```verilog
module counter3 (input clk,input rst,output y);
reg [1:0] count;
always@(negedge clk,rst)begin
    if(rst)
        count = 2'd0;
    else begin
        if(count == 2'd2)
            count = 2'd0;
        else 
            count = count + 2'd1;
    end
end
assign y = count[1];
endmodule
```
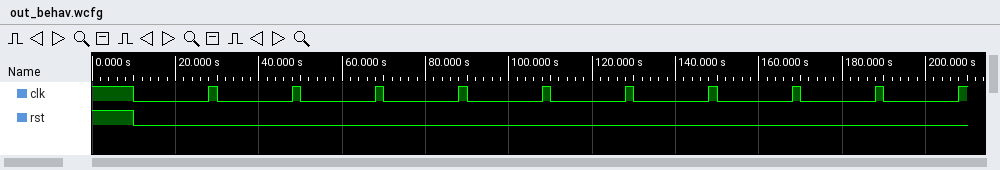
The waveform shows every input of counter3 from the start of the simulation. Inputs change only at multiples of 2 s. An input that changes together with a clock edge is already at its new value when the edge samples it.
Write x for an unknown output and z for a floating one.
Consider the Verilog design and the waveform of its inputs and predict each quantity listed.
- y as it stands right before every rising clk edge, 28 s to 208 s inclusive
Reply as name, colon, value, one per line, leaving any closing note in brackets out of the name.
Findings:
y as it stands right before every rising clk edge, 28 s to 208 s inclusive: 1 0 0 1 0 0 1 0 0 1
